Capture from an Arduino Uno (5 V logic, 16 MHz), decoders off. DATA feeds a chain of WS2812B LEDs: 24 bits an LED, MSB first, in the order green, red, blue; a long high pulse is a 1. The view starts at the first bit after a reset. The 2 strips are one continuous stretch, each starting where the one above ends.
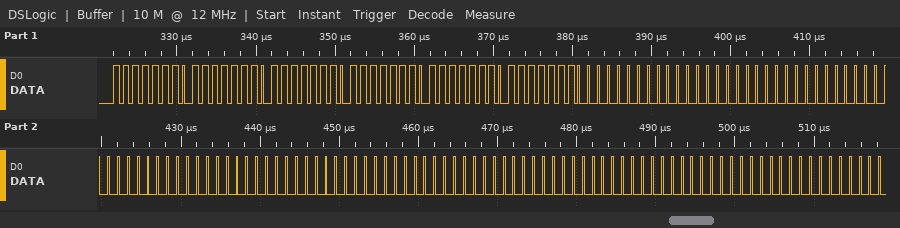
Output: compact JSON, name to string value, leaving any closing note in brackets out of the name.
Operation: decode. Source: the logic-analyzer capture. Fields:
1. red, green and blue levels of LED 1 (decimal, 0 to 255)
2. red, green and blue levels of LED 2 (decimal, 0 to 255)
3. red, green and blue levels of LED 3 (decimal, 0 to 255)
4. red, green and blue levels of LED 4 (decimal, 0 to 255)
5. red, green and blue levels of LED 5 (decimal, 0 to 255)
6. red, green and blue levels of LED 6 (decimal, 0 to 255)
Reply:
{"red, green and blue levels of LED 1": "254, 254, 254", "red, green and blue levels of LED 2": "254, 254, 254", "red, green and blue levels of LED 3": "0, 0, 0", "red, green and blue levels of LED 4": "0, 0, 0", "red, green and blue levels of LED 5": "0, 0, 0", "red, green and blue levels of LED 6": "0, 0, 0"}
